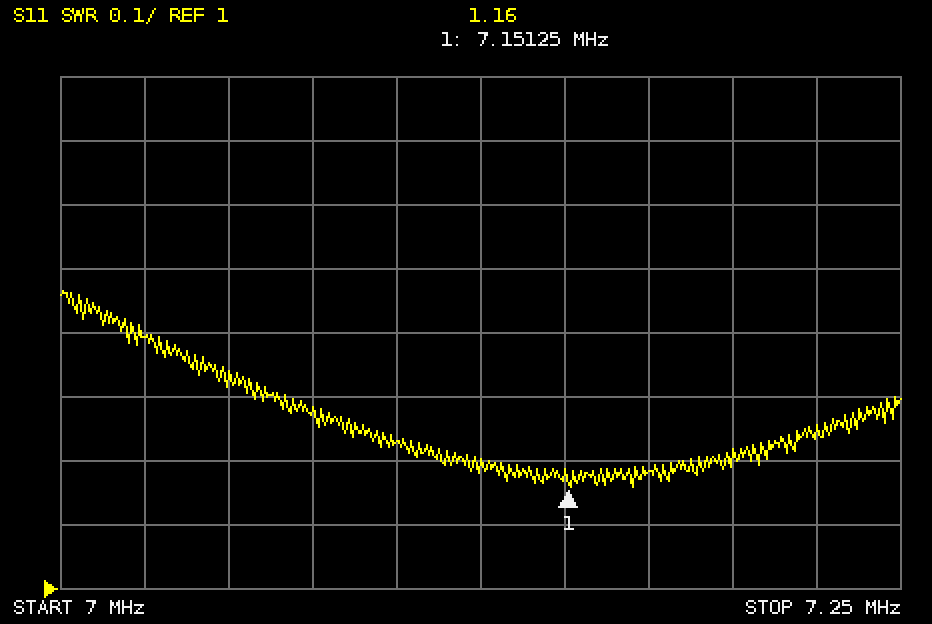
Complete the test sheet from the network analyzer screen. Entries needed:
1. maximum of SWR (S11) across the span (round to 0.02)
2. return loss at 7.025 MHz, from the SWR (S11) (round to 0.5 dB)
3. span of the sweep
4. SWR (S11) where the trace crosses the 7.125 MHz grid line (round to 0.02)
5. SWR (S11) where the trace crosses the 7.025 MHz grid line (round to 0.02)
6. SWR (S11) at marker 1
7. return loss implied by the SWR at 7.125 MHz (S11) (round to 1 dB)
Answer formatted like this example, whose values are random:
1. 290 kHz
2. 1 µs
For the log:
1. 1.46
2. 15.5 dB
3. 250 kHz
4. 1.20
5. 1.40
6. 1.16
7. 21 dB
